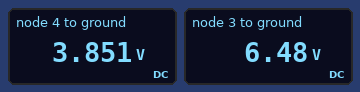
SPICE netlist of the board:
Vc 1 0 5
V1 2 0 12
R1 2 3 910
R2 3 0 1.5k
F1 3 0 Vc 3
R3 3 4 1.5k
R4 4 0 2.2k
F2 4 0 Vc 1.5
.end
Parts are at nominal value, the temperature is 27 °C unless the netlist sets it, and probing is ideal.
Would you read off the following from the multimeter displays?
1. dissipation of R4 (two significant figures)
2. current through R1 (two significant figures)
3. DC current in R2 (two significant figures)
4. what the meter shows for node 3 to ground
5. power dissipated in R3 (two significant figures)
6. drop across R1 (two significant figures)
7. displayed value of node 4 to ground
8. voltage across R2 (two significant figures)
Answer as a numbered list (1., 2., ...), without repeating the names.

1. 6.7 mW
2. 6.1 mA
3. 4.3 mA
4. 6.48 V
5. 4.6 mW
6. 5.5 V
7. 3.851 V
8. 6.5 V
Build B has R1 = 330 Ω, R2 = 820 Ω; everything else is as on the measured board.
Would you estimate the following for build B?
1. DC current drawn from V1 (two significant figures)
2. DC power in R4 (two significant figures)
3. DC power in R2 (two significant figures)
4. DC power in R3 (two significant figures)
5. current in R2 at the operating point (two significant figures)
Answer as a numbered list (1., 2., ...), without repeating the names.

1. 12 mA
2. 10 mW
3. 79 mW
4. 7.1 mW
5. 9.8 mA
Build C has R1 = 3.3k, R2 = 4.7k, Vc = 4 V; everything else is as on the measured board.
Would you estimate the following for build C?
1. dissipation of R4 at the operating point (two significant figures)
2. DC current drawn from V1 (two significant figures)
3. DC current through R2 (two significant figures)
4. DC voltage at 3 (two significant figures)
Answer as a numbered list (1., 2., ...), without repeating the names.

1. 3.4 mW
2. 2.2 mA
3. 980 µA
4. 4.6 V
